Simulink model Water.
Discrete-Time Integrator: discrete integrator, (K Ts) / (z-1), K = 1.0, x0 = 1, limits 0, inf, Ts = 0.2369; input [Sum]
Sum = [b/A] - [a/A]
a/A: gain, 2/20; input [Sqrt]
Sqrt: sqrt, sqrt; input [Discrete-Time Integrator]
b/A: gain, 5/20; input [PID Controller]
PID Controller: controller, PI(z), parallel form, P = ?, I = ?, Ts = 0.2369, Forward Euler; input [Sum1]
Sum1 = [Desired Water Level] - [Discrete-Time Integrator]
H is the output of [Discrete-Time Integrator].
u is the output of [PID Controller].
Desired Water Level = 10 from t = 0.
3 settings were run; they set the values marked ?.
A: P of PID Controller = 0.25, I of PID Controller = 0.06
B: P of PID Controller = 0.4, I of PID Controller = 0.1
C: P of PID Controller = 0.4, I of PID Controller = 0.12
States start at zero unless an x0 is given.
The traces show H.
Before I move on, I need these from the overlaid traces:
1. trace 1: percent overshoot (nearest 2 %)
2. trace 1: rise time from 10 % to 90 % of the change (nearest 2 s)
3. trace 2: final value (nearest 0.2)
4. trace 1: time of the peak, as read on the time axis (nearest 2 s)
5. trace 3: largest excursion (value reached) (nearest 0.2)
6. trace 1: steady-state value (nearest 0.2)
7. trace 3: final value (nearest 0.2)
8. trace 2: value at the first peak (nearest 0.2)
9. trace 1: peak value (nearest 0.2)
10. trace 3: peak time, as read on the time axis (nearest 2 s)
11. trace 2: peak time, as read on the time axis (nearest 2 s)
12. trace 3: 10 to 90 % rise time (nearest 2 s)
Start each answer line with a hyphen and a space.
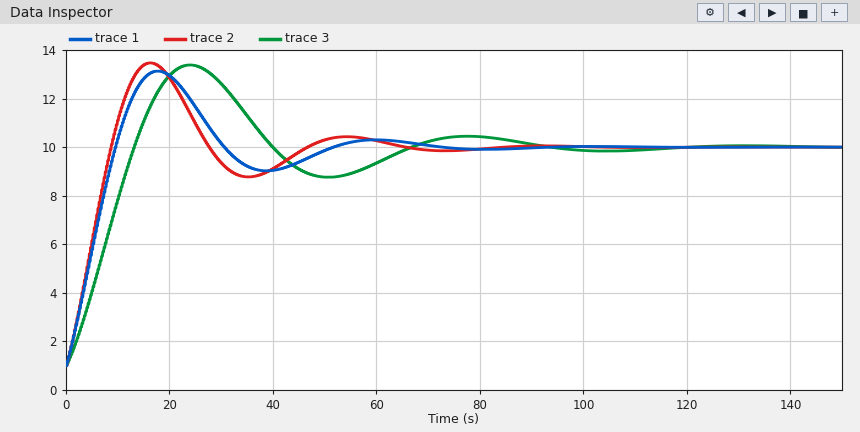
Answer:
- 34 %
- 8 s
- 10.0
- 18 s
- 13.4
- 10.0
- 10.0
- 13.4
- 13.2
- 24 s
- 16 s
- 10 s
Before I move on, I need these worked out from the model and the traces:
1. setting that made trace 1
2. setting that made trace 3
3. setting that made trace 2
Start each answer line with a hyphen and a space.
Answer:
- B
- A
- C
